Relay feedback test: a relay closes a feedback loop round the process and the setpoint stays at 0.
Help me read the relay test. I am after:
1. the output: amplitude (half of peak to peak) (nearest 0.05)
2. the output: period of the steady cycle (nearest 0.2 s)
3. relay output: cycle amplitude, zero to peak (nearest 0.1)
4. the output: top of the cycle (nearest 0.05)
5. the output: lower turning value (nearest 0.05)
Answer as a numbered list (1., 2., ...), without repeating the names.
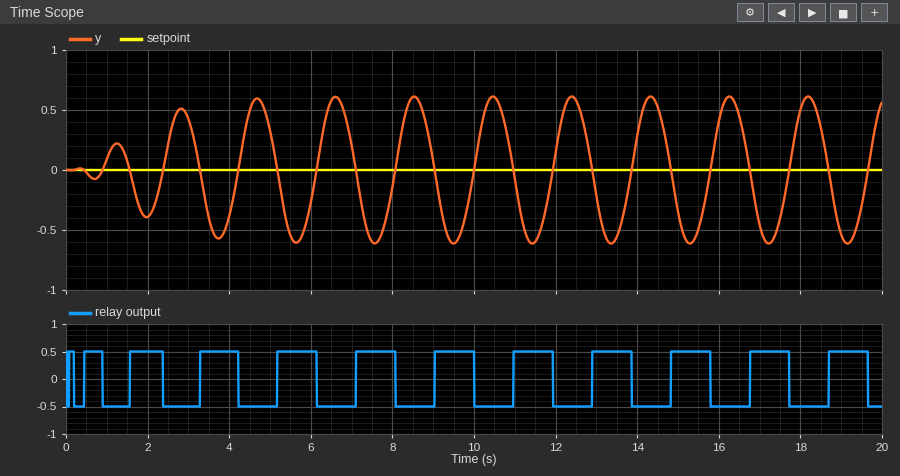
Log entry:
1. 0.60
2. 2.0 s
3. 0.5
4. 0.60
5. -0.60
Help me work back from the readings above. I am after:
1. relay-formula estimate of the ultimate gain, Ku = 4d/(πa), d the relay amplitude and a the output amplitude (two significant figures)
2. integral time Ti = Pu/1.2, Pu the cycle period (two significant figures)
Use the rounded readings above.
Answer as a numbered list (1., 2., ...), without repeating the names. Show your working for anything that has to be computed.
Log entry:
1. 4 × 0.5 / (π × 0.6) = 1.1
2. 2 / 1.2 = 1.7 s
